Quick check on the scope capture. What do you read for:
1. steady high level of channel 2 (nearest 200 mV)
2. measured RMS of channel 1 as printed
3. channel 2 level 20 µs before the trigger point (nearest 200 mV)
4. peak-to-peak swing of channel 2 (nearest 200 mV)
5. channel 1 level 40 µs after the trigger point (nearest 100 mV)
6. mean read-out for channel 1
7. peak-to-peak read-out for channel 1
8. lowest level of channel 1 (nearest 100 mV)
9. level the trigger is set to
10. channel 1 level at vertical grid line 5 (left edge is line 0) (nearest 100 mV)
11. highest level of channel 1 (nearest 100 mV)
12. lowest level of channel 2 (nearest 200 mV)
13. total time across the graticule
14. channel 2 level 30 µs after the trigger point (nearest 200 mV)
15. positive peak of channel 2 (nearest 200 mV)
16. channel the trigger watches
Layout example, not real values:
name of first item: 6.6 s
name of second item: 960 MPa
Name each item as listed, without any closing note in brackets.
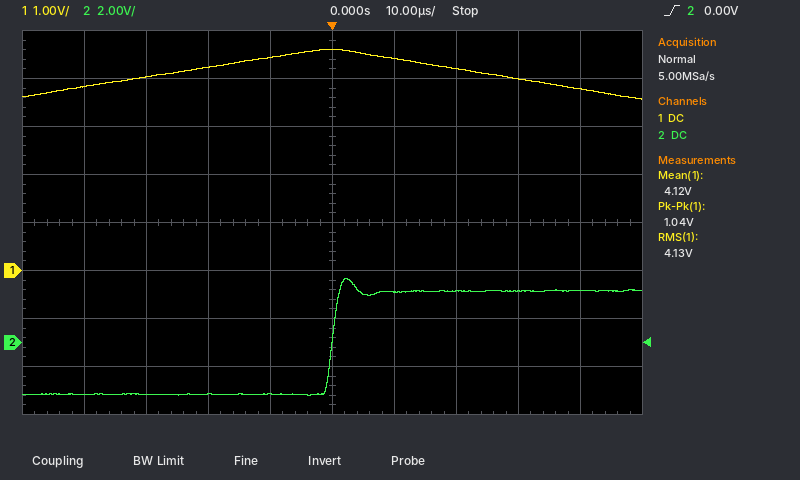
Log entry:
steady high level of channel 2: 2.2 V
measured RMS of channel 1 as printed: 4.13 V
channel 2 level 20 µs before the trigger point: -2.2 V
peak-to-peak swing of channel 2: 4.8 V
channel 1 level 40 µs after the trigger point: 3.8 V
mean read-out for channel 1: 4.12 V
peak-to-peak read-out for channel 1: 1.04 V
lowest level of channel 1: 3.6 V
level the trigger is set to: 0.00 V
channel 1 level at vertical grid line 5 (left edge is line 0): 4.6 V
highest level of channel 1: 4.6 V
lowest level of channel 2: -2.2 V
total time across the graticule: 100 µs
channel 2 level 30 µs after the trigger point: 2.2 V
positive peak of channel 2: 2.6 V
channel the trigger watches: channel 2
